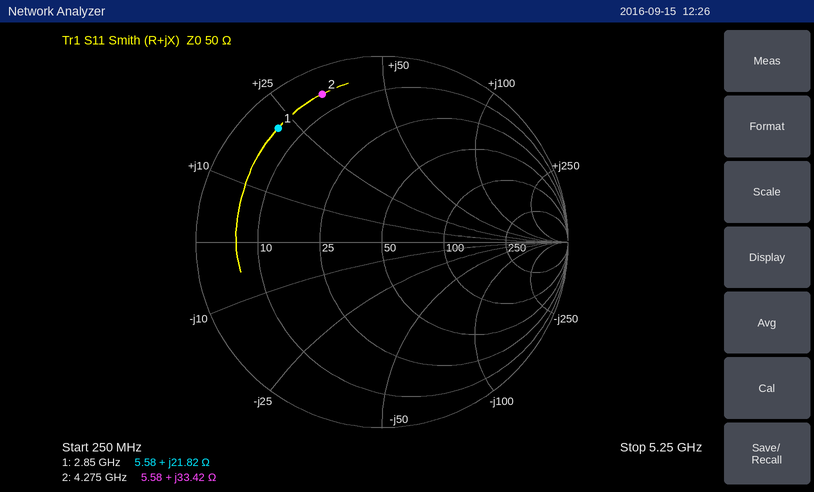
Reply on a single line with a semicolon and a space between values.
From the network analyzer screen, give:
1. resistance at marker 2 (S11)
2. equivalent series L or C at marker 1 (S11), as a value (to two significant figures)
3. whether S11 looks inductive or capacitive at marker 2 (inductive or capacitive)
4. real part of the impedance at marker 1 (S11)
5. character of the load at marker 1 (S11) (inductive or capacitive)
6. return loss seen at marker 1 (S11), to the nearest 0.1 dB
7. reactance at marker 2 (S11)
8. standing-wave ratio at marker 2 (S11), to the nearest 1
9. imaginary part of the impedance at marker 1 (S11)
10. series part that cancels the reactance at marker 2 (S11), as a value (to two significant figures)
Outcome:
5.58 Ω; 1.2 nH; inductive; 5.58 Ω; inductive; 1.6 dB; +33.42 Ω; 13; +21.82 Ω; 1.1 pF
